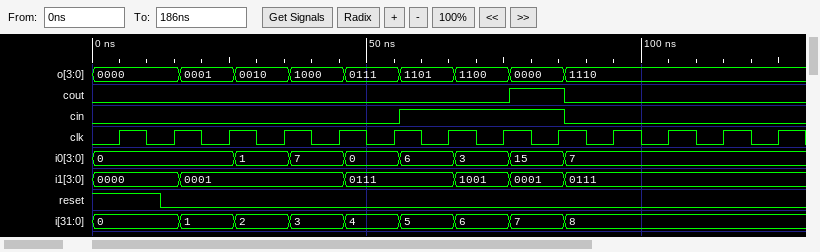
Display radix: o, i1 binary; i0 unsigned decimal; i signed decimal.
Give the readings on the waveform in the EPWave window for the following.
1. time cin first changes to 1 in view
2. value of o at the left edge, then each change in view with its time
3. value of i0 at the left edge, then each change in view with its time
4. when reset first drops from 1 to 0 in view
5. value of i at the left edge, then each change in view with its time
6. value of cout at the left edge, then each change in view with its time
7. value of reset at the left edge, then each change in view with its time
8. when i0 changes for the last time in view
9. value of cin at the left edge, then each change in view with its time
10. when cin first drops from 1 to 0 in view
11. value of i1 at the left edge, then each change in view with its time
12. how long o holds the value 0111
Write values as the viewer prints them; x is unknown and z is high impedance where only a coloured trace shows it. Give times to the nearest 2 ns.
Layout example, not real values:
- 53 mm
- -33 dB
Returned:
- 56 ns
- 0000, 0001 at 16 ns, 0010 at 26 ns, 1000 at 36 ns, 0111 at 46 ns, 1101 at 56 ns, 1100 at 66 ns, 0000 at 76 ns, 1110 at 86 ns
- 0, 1 at 26 ns, 7 at 36 ns, 0 at 46 ns, 6 at 56 ns, 3 at 66 ns, 15 at 76 ns, 7 at 86 ns
- 12 ns
- 0, 1 at 16 ns, 2 at 26 ns, 3 at 36 ns, 4 at 46 ns, 5 at 56 ns, 6 at 66 ns, 7 at 76 ns, 8 at 86 ns
- 0, 1 at 76 ns, 0 at 86 ns
- 1, 0 at 12 ns
- 86 ns
- 0, 1 at 56 ns, 0 at 86 ns
- 86 ns
- 0000, 0001 at 16 ns, 0111 at 46 ns, 1001 at 66 ns, 0001 at 76 ns, 0111 at 86 ns
- 10 ns
